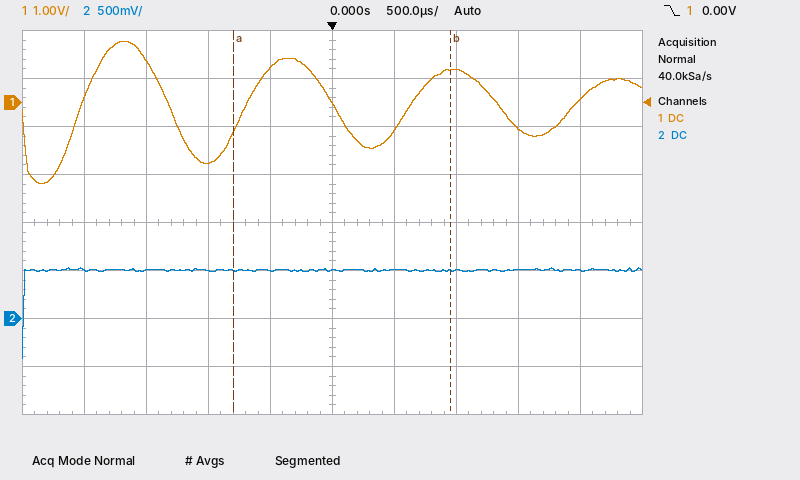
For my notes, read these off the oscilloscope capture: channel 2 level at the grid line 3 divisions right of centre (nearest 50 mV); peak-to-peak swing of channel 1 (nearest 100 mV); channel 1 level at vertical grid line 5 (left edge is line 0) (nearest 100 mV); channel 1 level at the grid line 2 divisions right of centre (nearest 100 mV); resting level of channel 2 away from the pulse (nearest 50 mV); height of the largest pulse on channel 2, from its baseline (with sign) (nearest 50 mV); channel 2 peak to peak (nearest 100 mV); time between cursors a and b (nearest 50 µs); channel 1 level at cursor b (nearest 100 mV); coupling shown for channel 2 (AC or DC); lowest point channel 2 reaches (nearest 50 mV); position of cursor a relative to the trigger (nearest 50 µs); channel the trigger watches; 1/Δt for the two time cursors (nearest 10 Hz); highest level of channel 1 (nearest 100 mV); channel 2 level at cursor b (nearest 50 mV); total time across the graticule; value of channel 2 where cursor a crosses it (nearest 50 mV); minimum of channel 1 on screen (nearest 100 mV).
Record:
500 mV
3.0 V
0.0 V
700 mV
500 mV
-900 mV
900 mV
1.75 ms
700 mV
DC
-400 mV
-800 µs
channel 1
570 Hz
1.3 V
500 mV
5 ms
500 mV
-1.7 V
